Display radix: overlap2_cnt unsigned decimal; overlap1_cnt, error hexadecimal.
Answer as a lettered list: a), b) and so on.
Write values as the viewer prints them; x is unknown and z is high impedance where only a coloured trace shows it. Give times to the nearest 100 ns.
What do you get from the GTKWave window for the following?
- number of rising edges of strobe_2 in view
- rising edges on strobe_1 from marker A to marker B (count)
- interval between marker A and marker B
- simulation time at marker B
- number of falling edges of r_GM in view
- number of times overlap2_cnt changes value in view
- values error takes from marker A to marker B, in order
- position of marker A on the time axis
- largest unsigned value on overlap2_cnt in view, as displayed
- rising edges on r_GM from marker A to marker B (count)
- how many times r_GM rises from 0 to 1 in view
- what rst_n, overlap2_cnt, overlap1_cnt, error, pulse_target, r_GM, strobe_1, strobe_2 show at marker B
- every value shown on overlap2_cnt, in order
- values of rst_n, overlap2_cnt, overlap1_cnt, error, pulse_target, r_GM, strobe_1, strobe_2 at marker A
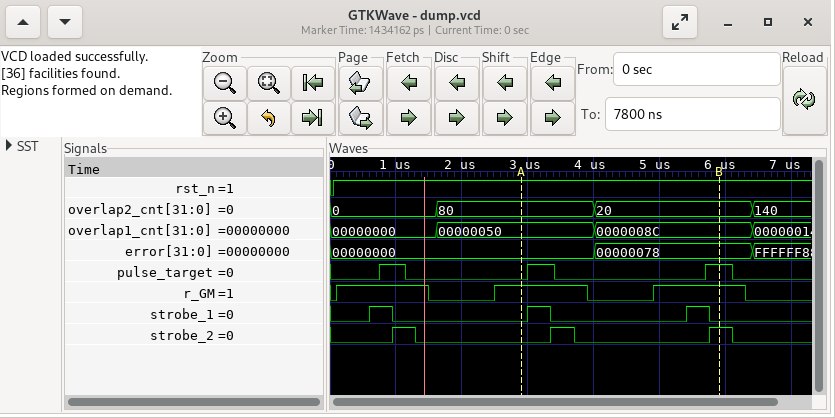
a) 3
b) 2
c) 3000 ns
d) 5900 ns
e) 3
f) 3
g) 00000000, 00000078
h) 2900 ns
i) 140
j) 1
k) 3
l) rst_n=1, overlap2_cnt=20, overlap1_cnt=0000008C, error=00000078, pulse_target=1, r_GM=1, strobe_1=0, strobe_2=1
m) 0, 80, 20, 140
n) rst_n=1, overlap2_cnt=80, overlap1_cnt=00000050, error=00000000, pulse_target=0, r_GM=1, strobe_1=0, strobe_2=0
